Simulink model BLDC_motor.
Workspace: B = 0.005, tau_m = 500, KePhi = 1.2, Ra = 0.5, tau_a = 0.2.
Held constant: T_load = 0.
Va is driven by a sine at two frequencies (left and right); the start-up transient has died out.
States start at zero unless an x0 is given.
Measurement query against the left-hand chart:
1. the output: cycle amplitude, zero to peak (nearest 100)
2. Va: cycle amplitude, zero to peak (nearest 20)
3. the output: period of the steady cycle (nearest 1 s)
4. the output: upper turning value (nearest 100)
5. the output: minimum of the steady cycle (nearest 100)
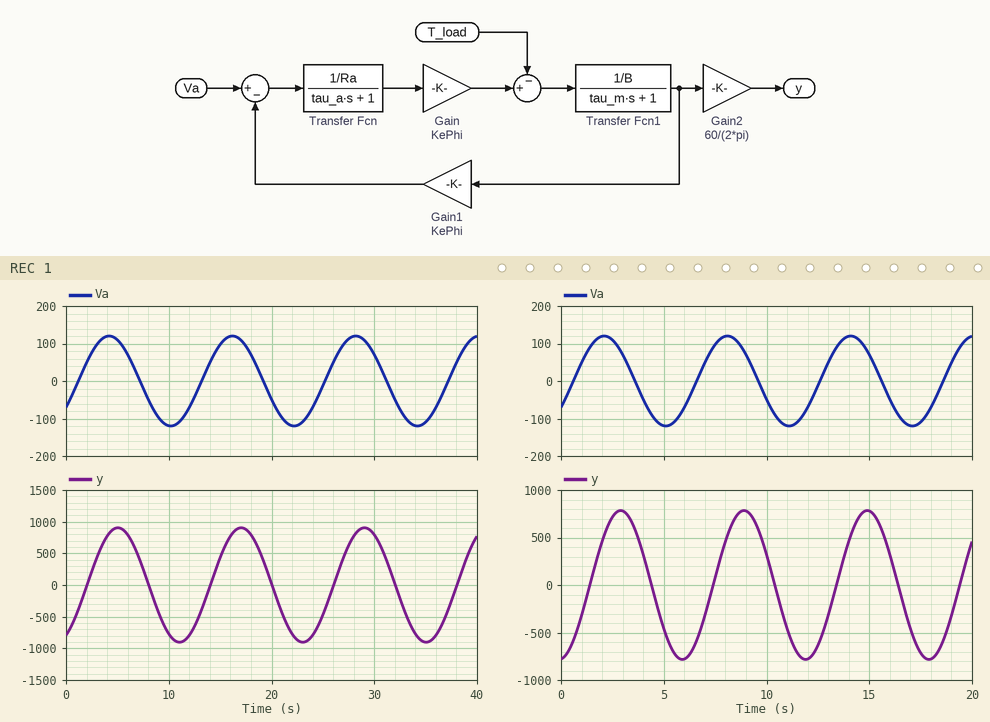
900
120
12 s
900
-900
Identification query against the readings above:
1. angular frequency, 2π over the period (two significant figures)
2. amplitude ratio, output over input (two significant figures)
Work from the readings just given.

0.52 rad/s
7.5
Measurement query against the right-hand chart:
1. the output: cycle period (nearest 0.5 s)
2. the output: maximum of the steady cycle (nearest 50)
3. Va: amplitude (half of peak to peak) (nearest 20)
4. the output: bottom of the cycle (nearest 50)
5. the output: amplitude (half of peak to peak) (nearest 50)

6.0 s
800
120
-800
800
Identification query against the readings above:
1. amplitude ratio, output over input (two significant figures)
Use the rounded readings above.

6.7
